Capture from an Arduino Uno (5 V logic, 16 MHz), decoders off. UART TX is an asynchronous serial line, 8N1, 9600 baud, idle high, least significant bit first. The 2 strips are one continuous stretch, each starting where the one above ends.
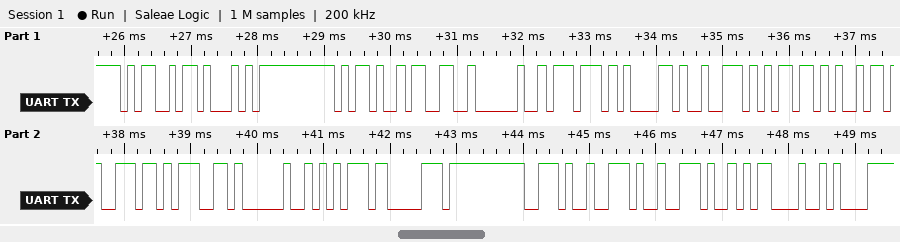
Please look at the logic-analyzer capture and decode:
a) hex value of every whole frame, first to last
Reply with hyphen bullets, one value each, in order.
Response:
- 4D 51 2D 33 20 77 61 72 6D 69 6E 67 20 75 70 2E 2E 2E 0D 0A
